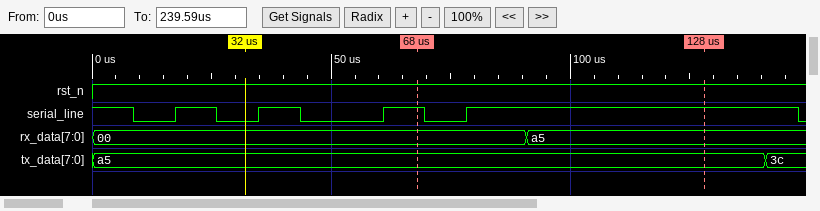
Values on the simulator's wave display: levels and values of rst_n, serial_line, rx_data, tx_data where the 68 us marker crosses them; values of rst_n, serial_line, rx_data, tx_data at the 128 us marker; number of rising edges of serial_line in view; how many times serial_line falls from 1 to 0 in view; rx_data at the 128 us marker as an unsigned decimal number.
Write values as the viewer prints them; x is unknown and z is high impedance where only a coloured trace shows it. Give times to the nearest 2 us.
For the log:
rst_n=1, serial_line=1, rx_data=00, tx_data=a5
rst_n=1, serial_line=1, rx_data=a5, tx_data=a5
4
5
165
